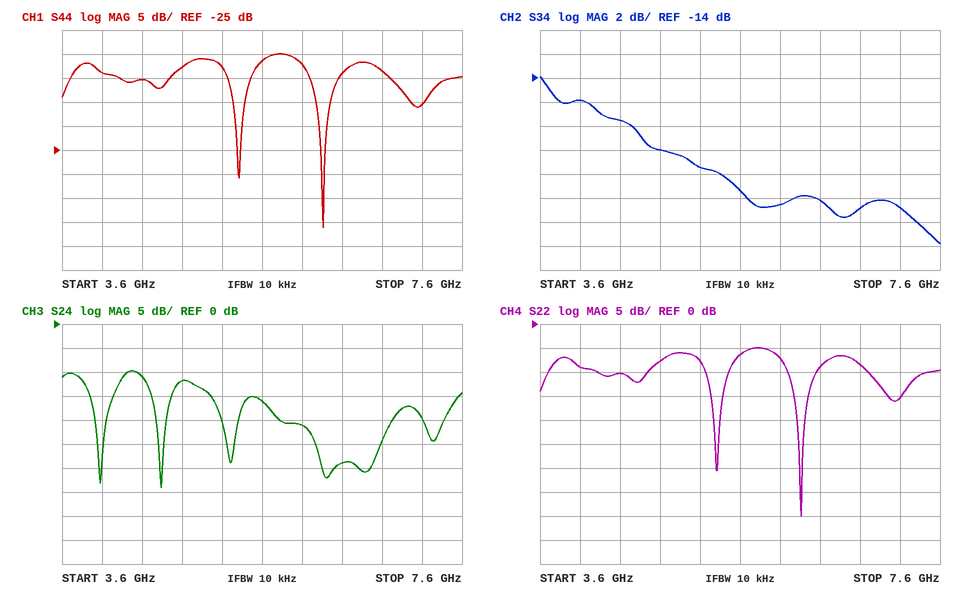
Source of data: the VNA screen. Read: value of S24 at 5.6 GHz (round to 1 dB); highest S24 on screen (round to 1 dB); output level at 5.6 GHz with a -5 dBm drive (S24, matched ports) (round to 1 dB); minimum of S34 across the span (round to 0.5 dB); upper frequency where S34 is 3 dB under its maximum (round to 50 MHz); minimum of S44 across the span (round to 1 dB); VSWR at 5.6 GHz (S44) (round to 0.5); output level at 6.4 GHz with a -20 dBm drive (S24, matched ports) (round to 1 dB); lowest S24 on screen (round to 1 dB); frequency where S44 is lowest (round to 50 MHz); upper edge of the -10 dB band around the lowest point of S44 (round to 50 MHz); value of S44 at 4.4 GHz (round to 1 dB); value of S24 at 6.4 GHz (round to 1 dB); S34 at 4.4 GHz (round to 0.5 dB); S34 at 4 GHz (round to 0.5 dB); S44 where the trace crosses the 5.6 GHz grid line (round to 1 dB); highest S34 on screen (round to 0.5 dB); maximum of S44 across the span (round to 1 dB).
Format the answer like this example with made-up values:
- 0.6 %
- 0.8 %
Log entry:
- -16 dB
- -10 dB
- -21 dBm
- -28.0 dB
- 4.20 GHz
- -41 dB
- 3.0
- -49 dBm
- -34 dB
- 6.20 GHz
- 6.35 GHz
- -10 dB
- -29 dB
- -17.5 dB
- -16.0 dB
- -6 dB
- -14.0 dB
- -5 dB
